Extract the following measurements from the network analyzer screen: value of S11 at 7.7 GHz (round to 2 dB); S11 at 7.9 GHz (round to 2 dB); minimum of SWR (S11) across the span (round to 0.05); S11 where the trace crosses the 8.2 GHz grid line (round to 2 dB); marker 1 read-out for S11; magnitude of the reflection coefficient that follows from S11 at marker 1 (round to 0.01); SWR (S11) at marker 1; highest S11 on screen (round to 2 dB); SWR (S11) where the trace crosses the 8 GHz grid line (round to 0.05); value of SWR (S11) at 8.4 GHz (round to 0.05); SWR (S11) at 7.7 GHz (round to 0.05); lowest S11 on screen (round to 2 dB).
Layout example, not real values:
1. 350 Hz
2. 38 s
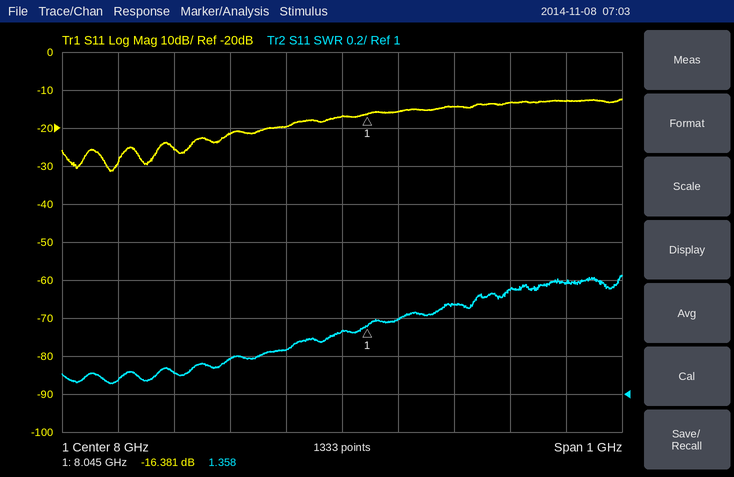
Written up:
1. -26 dB
2. -20 dB
3. 1.05
4. -14 dB
5. -16.381 dB
6. 0.15
7. 1.358
8. -12 dB
9. 1.35
10. 1.60
11. 1.10
12. -32 dB
